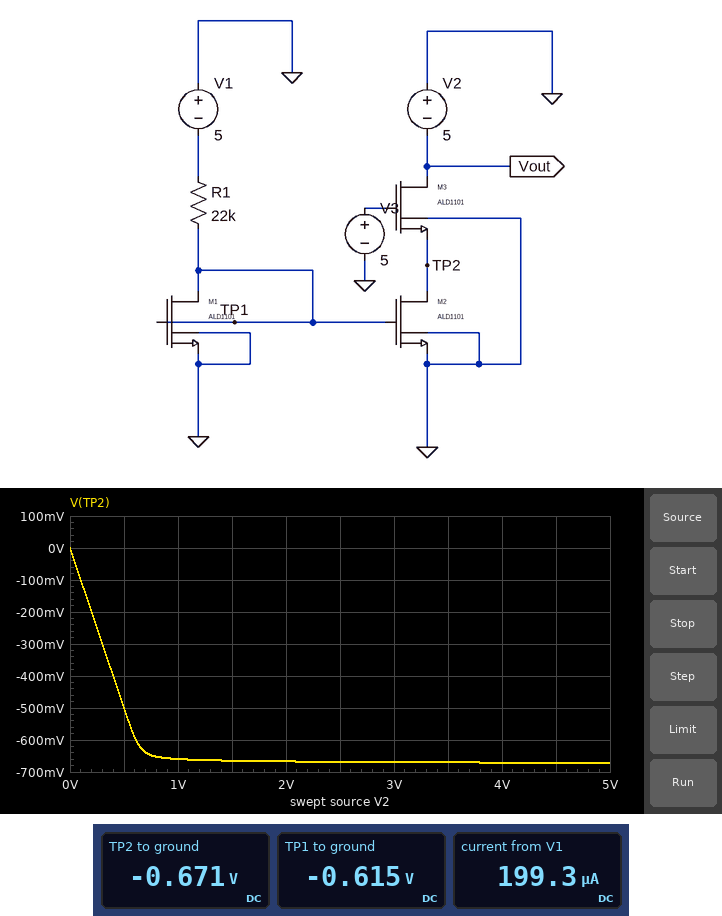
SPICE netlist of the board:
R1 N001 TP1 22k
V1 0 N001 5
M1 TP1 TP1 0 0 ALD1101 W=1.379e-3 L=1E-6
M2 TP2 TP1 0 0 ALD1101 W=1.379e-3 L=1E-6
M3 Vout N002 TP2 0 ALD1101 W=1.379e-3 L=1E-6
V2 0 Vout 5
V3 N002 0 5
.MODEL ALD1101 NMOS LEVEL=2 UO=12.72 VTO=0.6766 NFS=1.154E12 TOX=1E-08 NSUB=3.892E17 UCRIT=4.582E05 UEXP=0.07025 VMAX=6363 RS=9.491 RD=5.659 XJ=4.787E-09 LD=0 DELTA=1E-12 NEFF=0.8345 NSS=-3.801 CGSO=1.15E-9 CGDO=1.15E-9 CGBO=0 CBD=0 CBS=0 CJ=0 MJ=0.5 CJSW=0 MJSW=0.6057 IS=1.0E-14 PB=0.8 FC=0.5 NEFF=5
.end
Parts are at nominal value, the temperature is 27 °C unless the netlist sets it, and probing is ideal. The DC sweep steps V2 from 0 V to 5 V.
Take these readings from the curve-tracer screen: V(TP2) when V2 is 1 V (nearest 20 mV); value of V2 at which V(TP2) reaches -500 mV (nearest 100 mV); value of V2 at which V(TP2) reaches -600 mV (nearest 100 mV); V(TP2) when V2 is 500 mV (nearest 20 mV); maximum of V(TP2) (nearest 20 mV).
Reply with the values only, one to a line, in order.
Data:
-660 mV
500 mV
600 mV
-500 mV
0 V
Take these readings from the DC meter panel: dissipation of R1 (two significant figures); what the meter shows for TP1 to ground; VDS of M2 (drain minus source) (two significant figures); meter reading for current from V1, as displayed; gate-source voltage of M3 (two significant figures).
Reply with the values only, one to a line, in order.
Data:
870 µW
-0.615 V
-670 mV
199.3 µA
5.7 V
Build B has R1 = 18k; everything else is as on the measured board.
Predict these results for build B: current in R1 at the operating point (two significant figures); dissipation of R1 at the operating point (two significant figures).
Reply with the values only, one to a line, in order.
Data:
240 µA
1.1 mW
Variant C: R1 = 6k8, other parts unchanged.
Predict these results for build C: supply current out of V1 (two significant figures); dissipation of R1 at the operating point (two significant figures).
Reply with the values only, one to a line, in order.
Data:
640 µA
2.8 mW
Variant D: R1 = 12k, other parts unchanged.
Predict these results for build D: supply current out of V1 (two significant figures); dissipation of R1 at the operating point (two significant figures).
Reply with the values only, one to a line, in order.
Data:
360 µA
1.6 mW
